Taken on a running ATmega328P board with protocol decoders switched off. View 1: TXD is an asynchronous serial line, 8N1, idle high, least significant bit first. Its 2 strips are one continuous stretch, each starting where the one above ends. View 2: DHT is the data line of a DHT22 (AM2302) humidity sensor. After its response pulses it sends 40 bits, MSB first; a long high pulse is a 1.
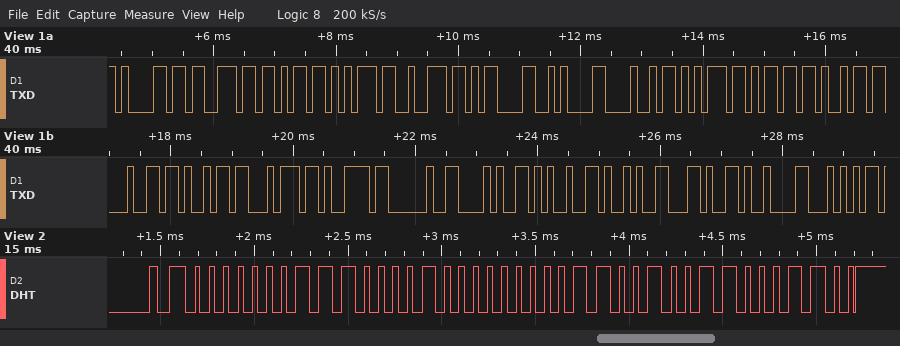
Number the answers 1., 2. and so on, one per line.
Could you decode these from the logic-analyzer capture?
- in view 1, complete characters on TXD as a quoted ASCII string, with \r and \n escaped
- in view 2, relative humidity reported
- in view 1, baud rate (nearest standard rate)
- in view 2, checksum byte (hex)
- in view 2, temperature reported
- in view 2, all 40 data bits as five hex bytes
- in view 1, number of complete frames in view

1. "askur\r\nHumidity (%),\tT"
2. 45.0 %
3. 9600 baud
4. 0x8C
5. 20.1 °C
6. 01 C2 00 C9 8C
7. 22
